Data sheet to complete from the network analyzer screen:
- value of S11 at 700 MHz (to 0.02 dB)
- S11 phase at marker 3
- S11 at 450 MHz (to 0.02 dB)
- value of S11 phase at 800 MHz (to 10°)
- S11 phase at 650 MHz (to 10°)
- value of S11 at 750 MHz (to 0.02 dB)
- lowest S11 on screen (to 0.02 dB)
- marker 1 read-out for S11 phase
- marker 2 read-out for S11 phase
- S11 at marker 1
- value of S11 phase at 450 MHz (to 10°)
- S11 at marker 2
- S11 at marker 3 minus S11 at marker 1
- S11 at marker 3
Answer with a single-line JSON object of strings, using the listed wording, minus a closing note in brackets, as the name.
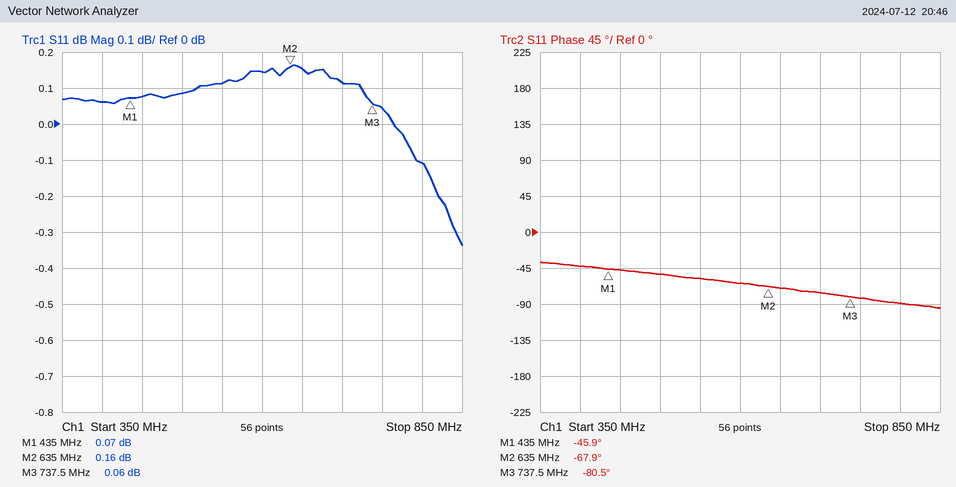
{"value of S11 at 700 MHz": "0.12 dB", "S11 phase at marker 3": "-80.5°", "S11 at 450 MHz": "0.08 dB", "value of S11 phase at 800 MHz": "-90°", "S11 phase at 650 MHz": "-70°", "value of S11 at 750 MHz": "0.04 dB", "lowest S11 on screen": "-0.34 dB", "marker 1 read-out for S11 phase": "-45.9°", "marker 2 read-out for S11 phase": "-67.9°", "S11 at marker 1": "0.07 dB", "value of S11 phase at 450 MHz": "-50°", "S11 at marker 2": "0.16 dB", "S11 at marker 3 minus S11 at marker 1": "-0.01 dB", "S11 at marker 3": "0.06 dB"}
